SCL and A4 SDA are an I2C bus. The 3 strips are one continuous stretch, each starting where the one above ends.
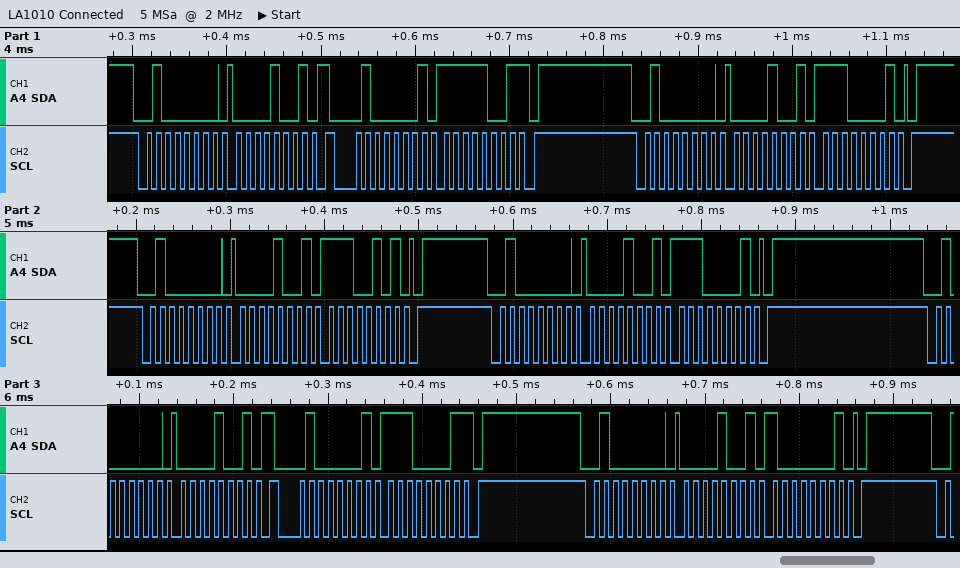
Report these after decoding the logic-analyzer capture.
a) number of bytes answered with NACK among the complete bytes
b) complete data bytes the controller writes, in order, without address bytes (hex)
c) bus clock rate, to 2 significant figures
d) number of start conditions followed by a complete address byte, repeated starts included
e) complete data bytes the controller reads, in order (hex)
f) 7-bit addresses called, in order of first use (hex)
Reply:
2
09 09 E1 09 E5 09 E1 09 09 81
100 kHz
8
F9 E1
0x20
